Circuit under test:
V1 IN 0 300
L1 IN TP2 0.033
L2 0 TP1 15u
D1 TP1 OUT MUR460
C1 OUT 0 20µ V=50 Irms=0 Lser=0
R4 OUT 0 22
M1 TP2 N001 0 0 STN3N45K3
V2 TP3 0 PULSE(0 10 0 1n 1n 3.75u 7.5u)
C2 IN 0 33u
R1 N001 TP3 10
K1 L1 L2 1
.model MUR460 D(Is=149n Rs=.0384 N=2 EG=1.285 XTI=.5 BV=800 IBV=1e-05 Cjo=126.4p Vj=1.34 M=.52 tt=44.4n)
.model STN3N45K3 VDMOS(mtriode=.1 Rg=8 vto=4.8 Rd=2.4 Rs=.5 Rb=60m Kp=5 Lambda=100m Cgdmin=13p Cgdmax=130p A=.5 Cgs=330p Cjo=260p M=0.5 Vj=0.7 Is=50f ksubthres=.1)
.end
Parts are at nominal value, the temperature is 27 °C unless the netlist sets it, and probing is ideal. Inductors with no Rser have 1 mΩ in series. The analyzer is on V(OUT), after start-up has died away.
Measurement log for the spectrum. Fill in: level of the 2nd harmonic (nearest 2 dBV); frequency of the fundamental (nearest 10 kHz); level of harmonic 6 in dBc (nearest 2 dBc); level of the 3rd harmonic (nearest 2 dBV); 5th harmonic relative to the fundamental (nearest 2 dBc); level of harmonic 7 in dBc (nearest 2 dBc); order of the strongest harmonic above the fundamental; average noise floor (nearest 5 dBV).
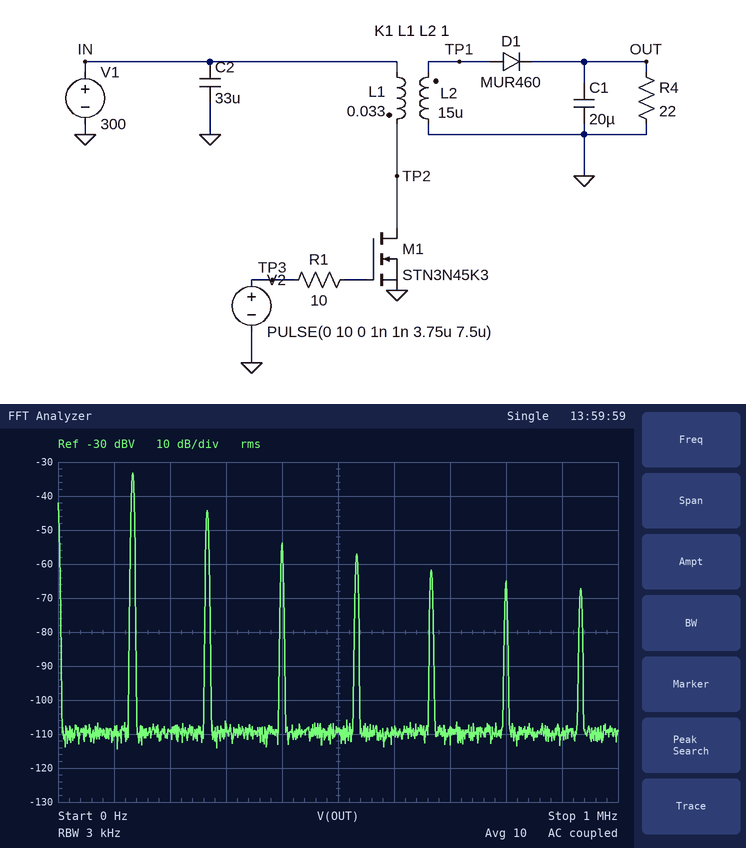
-44 dBV
130 kHz
-32 dBc
-54 dBV
-28 dBc
-34 dBc
2
-110 dBV
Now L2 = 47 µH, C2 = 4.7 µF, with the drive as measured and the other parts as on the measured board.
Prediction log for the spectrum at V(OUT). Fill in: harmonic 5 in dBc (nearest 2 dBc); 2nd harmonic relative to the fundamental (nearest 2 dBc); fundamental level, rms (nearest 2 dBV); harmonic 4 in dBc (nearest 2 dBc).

-30 dBc
-18 dBc
-30 dBV
-28 dBc
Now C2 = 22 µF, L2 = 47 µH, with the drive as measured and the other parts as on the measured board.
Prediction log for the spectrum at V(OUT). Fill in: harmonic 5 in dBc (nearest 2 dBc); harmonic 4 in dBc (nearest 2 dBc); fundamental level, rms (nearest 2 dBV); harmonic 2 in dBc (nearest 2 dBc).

-30 dBc
-28 dBc
-30 dBV
-18 dBc
